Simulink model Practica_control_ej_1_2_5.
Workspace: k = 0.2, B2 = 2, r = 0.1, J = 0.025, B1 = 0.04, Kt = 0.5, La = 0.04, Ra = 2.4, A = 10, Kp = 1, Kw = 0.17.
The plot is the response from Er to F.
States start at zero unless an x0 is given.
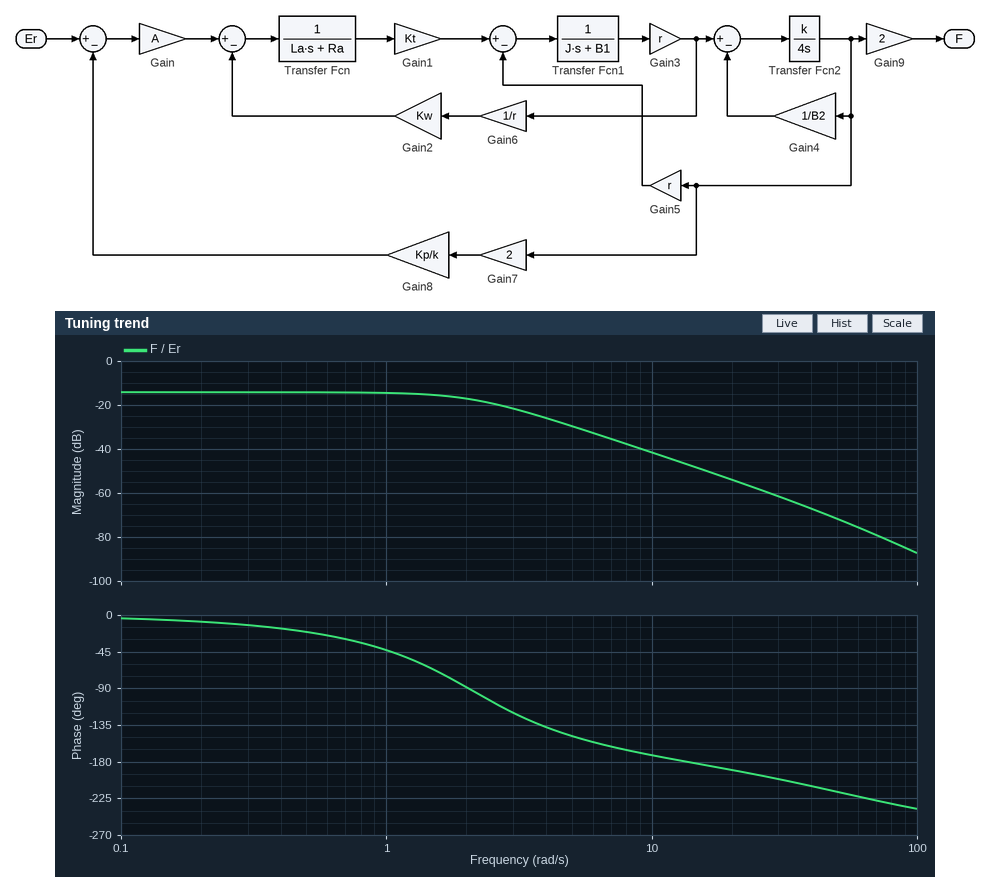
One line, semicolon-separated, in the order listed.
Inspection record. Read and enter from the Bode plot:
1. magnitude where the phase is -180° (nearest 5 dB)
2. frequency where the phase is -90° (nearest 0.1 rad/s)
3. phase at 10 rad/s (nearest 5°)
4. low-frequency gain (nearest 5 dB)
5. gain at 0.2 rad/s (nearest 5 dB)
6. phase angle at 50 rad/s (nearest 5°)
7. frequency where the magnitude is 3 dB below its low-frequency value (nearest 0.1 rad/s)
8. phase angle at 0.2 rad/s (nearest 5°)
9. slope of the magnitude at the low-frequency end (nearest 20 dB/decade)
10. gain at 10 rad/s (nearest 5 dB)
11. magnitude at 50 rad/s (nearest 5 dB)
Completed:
-45 dB; 2.0 rad/s; -170°; -15 dB; -15 dB; -215°; 2.0 rad/s; -10°; 0 dB/decade; -40 dB; -70 dB
